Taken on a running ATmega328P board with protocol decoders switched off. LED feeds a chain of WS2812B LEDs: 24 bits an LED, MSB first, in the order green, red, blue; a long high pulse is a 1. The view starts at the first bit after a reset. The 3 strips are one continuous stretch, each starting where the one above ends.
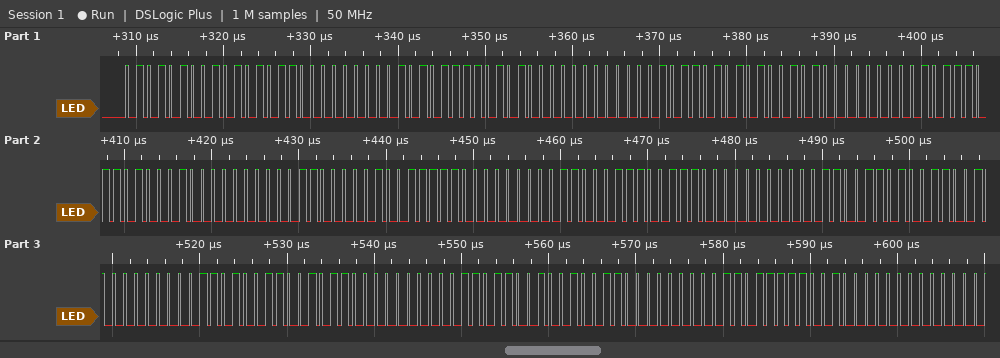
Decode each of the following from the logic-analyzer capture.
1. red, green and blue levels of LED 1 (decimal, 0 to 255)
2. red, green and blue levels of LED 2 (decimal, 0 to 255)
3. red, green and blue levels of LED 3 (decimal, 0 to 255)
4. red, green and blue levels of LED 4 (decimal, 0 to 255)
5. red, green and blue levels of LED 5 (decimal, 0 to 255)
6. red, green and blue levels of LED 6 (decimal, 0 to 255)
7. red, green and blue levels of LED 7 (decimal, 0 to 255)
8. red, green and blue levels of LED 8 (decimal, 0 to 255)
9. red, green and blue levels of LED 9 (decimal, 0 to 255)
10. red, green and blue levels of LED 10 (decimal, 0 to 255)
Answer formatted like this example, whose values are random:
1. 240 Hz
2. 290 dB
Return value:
1. 171, 84, 0
2. 168, 87, 0
3. 165, 90, 0
4. 162, 93, 0
5. 159, 96, 0
6. 156, 99, 0
7. 153, 102, 0
8. 150, 105, 0
9. 147, 108, 0
10. 144, 111, 0
